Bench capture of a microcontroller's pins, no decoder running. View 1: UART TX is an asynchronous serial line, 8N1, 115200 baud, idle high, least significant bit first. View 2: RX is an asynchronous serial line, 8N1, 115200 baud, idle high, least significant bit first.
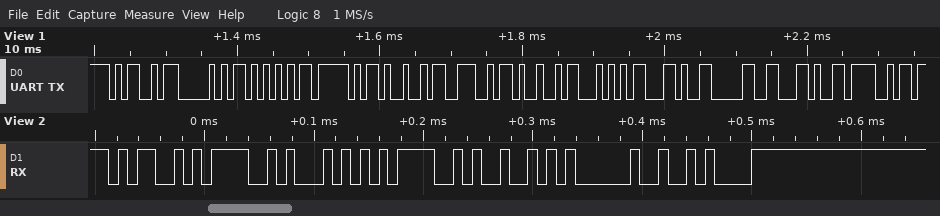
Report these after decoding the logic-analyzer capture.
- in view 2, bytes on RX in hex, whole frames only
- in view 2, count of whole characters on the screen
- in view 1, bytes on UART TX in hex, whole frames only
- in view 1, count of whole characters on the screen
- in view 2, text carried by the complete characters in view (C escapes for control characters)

4D 4F 54 4F 52 20 0A
7
0x4D 0x50 0x55 0x5F 0x49 0x4E 0x49 0x54 0x2C 0x30 0x2C 0x4F
12
"MOTOR \n"
